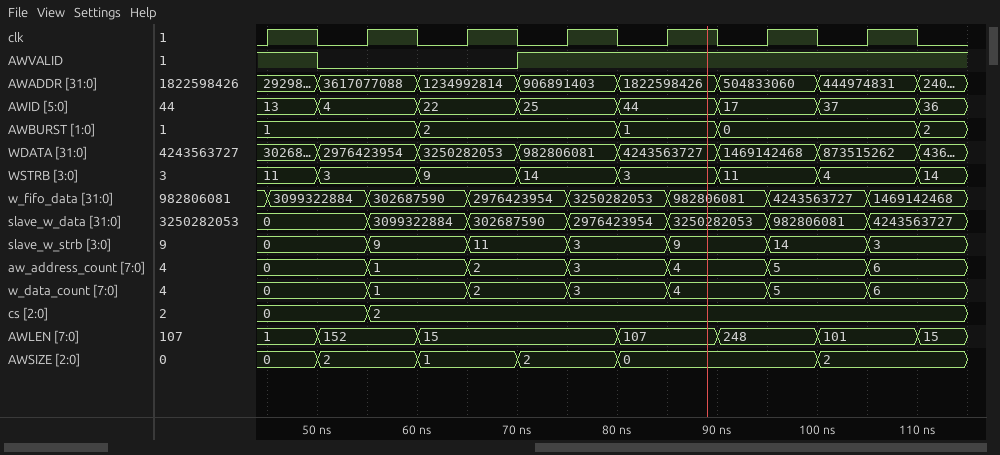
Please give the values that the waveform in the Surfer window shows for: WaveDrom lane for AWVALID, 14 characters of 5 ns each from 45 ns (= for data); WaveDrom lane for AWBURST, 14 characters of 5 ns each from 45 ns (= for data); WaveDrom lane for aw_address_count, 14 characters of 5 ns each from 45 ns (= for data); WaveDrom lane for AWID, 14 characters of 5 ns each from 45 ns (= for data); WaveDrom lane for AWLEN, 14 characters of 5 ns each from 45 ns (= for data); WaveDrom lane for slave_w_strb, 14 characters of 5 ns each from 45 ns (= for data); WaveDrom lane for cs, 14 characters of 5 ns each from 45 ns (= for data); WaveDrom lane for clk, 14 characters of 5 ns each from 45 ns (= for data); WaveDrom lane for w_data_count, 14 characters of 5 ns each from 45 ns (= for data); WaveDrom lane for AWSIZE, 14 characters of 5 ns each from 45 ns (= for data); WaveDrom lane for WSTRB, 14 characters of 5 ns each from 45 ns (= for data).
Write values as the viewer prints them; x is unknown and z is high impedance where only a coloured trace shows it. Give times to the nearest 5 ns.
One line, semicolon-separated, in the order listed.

{name: 'AWVALID', wave: '10...1........'}; {name: 'AWBURST', wave: '=..=...=.=...=', data: '1 2 1 0 2'}; {name: 'aw_address_count', wave: '=.=.=.=.=.=.=.', data: '0 1 2 3 4 5 6'}; {name: 'AWID', wave: '==.=.=.=.=.=.=', data: '13 4 22 25 44 17 37 36'}; {name: 'AWLEN', wave: '==.=...=.=.=.=', data: '1 152 15 107 248 101 15'}; {name: 'slave_w_strb', wave: '=.=.=.=.=.=.=.', data: '0 9 11 3 9 14 3'}; {name: 'cs', wave: '=.=...........', data: '0 2'}; {name: 'clk', wave: '10101010101010'}; {name: 'w_data_count', wave: '=.=.=.=.=.=.=.', data: '0 1 2 3 4 5 6'}; {name: 'AWSIZE', wave: '==.=.=.=...=..', data: '0 2 1 2 0 2'}; {name: 'WSTRB', wave: '==.=.=.=.=.=.=', data: '11 3 9 14 3 11 4 14'}
